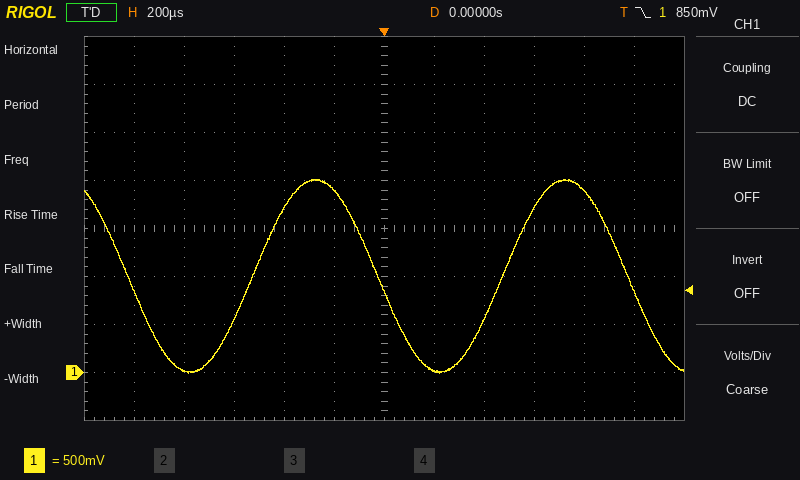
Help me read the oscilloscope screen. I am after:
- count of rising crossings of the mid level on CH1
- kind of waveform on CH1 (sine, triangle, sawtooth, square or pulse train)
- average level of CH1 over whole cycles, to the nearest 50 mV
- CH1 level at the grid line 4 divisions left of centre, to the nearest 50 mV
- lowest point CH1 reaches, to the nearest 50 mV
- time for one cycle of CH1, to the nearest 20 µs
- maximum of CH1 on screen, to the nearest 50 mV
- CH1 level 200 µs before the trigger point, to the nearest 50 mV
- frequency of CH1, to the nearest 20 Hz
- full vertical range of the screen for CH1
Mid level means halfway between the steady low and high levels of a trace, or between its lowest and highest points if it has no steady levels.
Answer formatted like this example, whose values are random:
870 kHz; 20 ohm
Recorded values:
2; sine; 1.00 V; 0 mV; 0 mV; 1.00 ms; 2.00 V; 1.90 V; 1.00 kHz; 4 V
